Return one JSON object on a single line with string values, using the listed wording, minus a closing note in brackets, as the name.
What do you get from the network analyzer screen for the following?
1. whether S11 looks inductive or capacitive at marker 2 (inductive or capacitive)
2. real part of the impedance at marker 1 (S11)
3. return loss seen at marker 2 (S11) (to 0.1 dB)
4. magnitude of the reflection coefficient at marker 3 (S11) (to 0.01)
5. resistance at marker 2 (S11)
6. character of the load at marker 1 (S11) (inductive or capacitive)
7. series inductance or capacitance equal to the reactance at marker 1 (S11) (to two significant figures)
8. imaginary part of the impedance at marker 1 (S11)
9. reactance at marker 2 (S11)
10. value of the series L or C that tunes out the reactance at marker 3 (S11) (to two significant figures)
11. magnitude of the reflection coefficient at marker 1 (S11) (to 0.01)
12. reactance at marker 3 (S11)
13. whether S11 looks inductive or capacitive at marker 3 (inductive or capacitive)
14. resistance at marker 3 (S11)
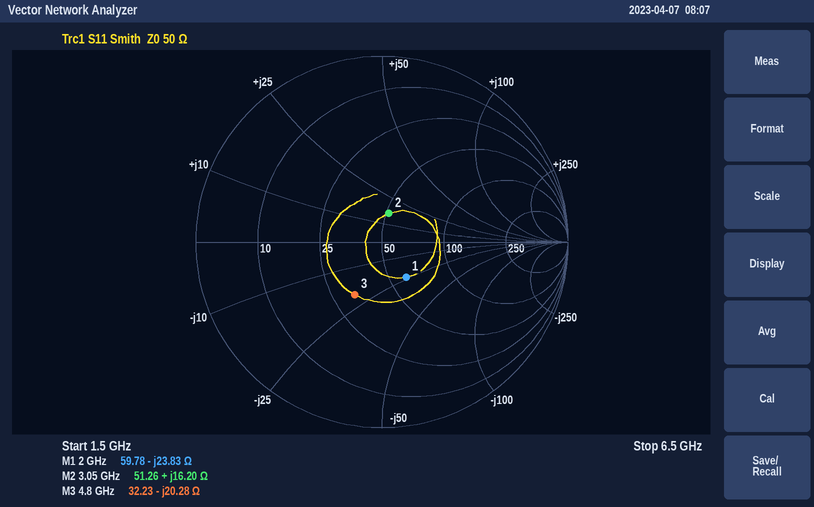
{"whether S11 looks inductive or capacitive at marker 2": "inductive", "real part of the impedance at marker 1": "59.78 Ω", "return loss seen at marker 2 (S11)": "16.0 dB", "magnitude of the reflection coefficient at marker 3 (S11)": "0.32", "resistance at marker 2": "51.26 Ω", "character of the load at marker 1 (S11)": "capacitive", "series inductance or capacitance equal to the reactance at marker 1 (S11)": "3.3 pF", "imaginary part of the impedance at marker 1": "-23.83 Ω", "reactance at marker 2": "+16.20 Ω", "value of the series L or C that tunes out the reactance at marker 3 (S11)": "670 pH", "magnitude of the reflection coefficient at marker 1 (S11)": "0.23", "reactance at marker 3": "-20.28 Ω", "whether S11 looks inductive or capacitive at marker 3": "capacitive", "resistance at marker 3": "32.23 Ω"}
